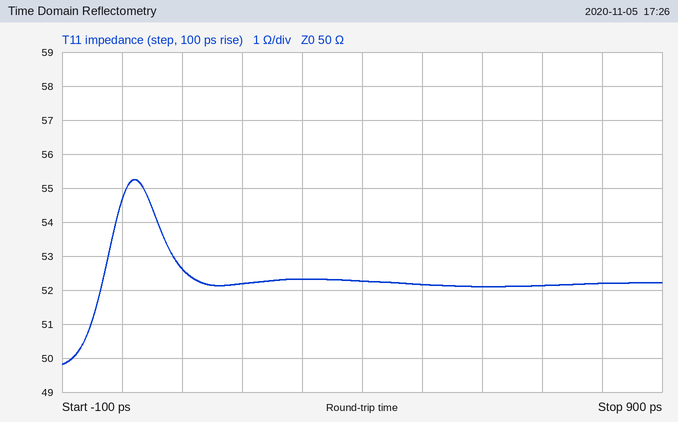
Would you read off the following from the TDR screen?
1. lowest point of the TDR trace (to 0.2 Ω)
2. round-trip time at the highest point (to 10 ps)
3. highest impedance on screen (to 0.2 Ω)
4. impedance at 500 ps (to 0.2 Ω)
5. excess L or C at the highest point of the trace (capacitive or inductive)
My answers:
49.8 Ω
20 ps
55.2 Ω
52.2 Ω
inductive
